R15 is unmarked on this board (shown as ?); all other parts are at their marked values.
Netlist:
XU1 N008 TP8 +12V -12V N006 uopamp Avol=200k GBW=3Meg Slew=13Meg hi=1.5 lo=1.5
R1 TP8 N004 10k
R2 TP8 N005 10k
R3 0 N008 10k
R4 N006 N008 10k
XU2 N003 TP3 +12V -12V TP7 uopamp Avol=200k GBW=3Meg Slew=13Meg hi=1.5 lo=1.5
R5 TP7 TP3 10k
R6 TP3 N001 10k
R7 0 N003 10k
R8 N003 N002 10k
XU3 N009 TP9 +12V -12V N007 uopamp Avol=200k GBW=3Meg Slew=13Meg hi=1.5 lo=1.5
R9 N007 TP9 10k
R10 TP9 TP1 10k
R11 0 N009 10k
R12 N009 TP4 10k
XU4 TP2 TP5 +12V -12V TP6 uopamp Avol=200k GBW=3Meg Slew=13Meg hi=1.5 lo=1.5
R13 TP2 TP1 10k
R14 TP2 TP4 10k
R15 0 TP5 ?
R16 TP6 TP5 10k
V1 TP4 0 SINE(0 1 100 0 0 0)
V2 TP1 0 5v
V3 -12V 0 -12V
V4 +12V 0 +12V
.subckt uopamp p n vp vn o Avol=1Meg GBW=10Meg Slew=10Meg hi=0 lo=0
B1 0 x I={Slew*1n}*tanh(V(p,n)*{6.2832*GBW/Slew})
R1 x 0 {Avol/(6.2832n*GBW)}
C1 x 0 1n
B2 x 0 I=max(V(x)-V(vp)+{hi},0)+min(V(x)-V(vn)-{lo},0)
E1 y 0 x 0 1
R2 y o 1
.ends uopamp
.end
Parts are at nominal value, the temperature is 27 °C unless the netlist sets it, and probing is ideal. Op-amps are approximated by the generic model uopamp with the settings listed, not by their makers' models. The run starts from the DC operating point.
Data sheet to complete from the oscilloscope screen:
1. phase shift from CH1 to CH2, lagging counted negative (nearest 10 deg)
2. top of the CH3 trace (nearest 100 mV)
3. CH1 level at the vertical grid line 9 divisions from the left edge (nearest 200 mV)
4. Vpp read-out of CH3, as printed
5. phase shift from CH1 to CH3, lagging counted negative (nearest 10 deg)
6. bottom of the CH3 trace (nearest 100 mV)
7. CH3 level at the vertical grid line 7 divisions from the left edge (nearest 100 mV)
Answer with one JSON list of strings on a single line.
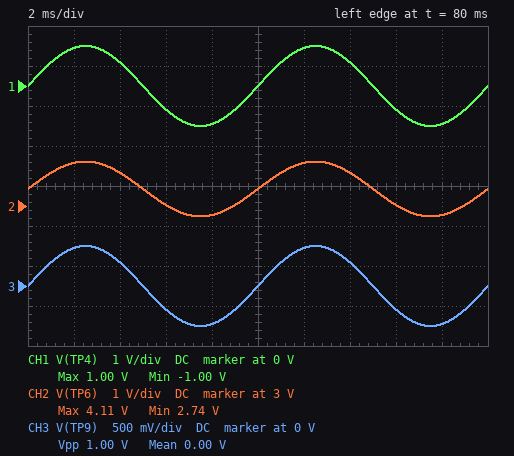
["0 deg", "500 mV", "-1.0 V", "1.00 V", "0 deg", "-500 mV", "300 mV"]
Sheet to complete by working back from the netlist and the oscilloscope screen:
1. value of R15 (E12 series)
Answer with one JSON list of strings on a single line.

["27 kΩ"]
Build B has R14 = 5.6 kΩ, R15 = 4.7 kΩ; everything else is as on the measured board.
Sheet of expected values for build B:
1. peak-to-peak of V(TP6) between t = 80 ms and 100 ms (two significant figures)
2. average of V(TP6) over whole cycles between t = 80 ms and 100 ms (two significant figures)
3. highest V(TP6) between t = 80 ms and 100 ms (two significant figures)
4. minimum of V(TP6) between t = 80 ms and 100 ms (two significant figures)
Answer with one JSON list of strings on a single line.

["4.0 V", "5.6 V", "7.6 V", "3.6 V"]
